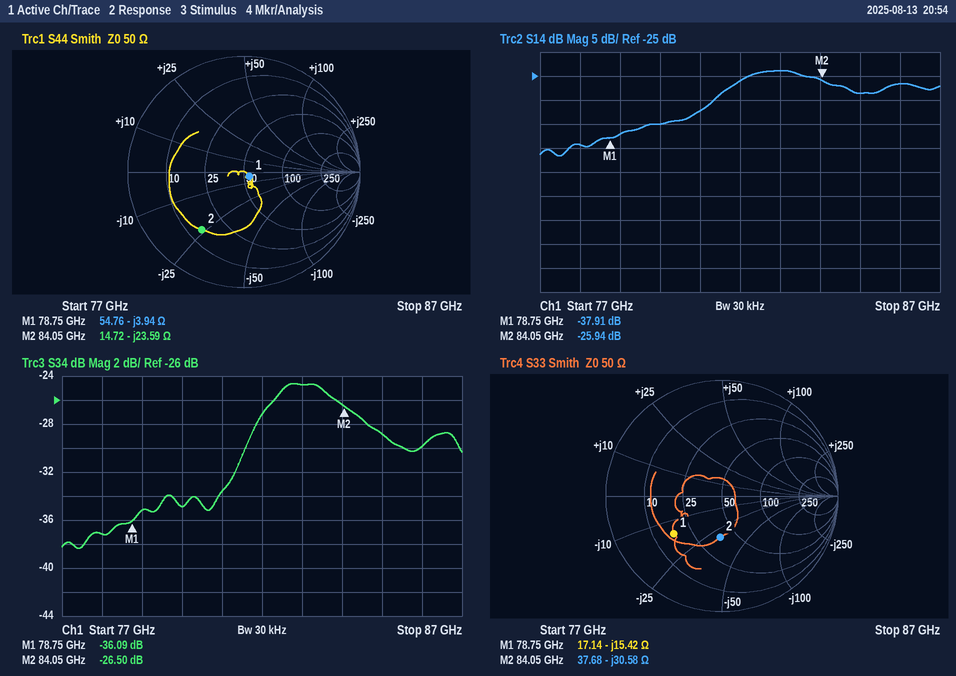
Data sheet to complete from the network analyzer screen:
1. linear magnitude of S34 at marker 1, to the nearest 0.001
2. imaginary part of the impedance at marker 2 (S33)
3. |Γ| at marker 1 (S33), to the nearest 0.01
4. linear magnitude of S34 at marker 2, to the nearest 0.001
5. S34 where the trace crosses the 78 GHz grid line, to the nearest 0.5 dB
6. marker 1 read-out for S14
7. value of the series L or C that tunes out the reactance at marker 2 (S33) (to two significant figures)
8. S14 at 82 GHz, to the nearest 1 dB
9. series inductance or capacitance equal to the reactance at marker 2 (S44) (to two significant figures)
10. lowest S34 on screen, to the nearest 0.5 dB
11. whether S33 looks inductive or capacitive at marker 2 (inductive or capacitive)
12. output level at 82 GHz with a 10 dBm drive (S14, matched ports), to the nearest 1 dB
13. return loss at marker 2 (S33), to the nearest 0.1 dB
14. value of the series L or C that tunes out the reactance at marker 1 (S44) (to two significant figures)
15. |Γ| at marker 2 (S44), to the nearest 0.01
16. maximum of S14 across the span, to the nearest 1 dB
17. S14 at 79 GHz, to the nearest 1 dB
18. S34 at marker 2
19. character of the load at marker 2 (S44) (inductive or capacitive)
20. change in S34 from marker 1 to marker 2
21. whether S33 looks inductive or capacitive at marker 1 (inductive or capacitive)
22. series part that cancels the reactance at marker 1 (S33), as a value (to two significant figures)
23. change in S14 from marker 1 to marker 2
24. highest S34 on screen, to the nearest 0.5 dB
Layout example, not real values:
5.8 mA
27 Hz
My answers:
0.016
-30.58 Ω
0.53
0.047
-37.0 dB
-37.91 dB
58 pH
-26 dB
80 fF
-38.5 dB
capacitive
-16 dBm
9.0 dB
8.0 pH
0.62
-24 dB
-37 dB
-26.50 dB
capacitive
9.59 dB
capacitive
31 pH
11.97 dB
-24.5 dB
